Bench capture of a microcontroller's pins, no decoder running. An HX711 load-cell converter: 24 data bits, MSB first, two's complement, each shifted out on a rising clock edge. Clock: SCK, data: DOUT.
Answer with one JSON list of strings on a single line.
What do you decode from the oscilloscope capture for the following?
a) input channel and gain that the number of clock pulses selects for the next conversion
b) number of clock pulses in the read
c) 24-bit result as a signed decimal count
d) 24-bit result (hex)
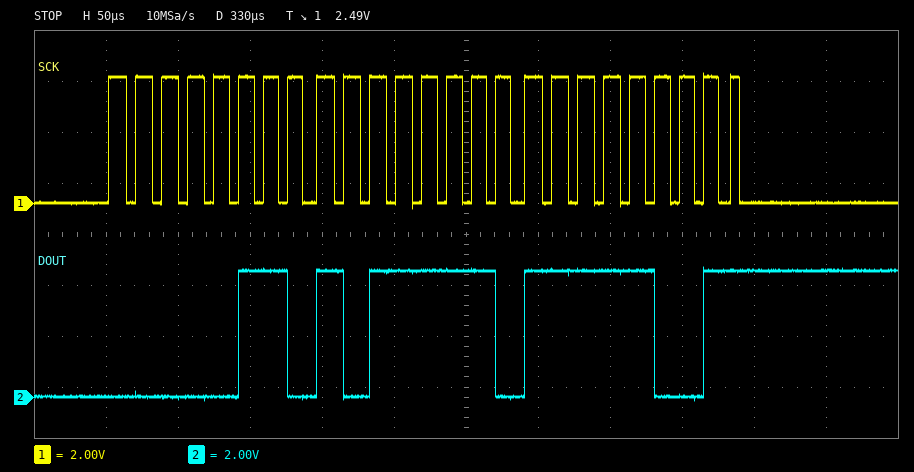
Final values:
["channel A, gain 128", "25", "442105", "0x06BEF9"]
